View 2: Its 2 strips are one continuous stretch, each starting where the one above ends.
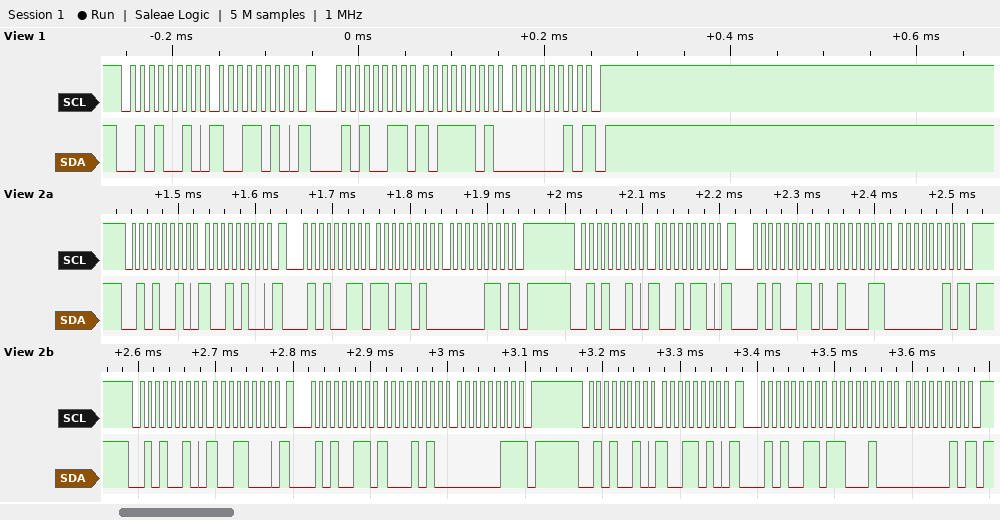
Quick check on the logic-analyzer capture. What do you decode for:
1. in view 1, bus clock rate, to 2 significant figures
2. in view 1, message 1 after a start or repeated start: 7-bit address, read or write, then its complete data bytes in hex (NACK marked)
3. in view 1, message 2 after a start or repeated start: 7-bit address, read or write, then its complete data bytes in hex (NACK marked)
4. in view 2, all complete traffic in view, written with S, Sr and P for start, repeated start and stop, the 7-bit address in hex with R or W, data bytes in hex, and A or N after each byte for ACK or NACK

100 kHz
0x29 write: 9A
0x29 read: BD 02 NACK
S 29W A 94 A Sr 29R A DA A 06 N P S 29W A 96 A Sr 29R A 23 A 02 N P S 29W A 98 A Sr 29R A 8A A 03 N P S 29W A 9A A Sr 29R A C4 A 02 N P
